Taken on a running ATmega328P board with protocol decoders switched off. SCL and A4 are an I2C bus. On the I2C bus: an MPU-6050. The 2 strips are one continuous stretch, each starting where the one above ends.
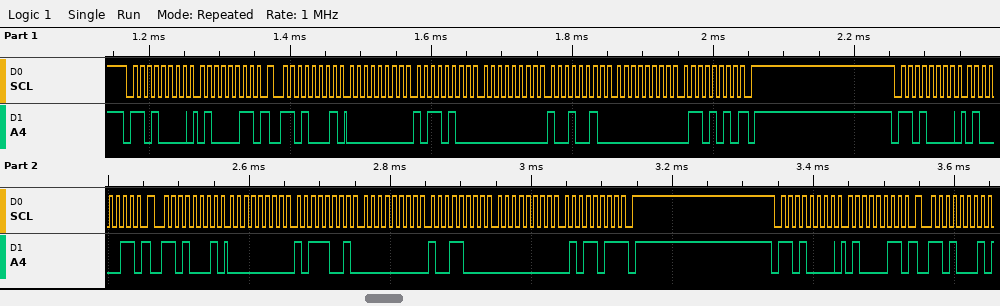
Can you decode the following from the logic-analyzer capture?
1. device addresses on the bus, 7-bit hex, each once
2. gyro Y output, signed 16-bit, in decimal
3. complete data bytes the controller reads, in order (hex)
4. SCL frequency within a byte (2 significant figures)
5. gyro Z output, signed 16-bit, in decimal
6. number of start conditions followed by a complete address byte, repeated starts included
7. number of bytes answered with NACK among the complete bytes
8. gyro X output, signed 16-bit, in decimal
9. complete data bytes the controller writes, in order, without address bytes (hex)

0x68
146
00 B4 00 92 00 6A 00 B9 00 98 00 5B
100 kHz
106
6
2
180
43 43 43
